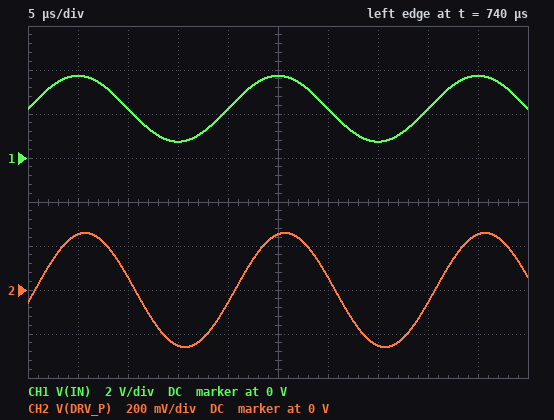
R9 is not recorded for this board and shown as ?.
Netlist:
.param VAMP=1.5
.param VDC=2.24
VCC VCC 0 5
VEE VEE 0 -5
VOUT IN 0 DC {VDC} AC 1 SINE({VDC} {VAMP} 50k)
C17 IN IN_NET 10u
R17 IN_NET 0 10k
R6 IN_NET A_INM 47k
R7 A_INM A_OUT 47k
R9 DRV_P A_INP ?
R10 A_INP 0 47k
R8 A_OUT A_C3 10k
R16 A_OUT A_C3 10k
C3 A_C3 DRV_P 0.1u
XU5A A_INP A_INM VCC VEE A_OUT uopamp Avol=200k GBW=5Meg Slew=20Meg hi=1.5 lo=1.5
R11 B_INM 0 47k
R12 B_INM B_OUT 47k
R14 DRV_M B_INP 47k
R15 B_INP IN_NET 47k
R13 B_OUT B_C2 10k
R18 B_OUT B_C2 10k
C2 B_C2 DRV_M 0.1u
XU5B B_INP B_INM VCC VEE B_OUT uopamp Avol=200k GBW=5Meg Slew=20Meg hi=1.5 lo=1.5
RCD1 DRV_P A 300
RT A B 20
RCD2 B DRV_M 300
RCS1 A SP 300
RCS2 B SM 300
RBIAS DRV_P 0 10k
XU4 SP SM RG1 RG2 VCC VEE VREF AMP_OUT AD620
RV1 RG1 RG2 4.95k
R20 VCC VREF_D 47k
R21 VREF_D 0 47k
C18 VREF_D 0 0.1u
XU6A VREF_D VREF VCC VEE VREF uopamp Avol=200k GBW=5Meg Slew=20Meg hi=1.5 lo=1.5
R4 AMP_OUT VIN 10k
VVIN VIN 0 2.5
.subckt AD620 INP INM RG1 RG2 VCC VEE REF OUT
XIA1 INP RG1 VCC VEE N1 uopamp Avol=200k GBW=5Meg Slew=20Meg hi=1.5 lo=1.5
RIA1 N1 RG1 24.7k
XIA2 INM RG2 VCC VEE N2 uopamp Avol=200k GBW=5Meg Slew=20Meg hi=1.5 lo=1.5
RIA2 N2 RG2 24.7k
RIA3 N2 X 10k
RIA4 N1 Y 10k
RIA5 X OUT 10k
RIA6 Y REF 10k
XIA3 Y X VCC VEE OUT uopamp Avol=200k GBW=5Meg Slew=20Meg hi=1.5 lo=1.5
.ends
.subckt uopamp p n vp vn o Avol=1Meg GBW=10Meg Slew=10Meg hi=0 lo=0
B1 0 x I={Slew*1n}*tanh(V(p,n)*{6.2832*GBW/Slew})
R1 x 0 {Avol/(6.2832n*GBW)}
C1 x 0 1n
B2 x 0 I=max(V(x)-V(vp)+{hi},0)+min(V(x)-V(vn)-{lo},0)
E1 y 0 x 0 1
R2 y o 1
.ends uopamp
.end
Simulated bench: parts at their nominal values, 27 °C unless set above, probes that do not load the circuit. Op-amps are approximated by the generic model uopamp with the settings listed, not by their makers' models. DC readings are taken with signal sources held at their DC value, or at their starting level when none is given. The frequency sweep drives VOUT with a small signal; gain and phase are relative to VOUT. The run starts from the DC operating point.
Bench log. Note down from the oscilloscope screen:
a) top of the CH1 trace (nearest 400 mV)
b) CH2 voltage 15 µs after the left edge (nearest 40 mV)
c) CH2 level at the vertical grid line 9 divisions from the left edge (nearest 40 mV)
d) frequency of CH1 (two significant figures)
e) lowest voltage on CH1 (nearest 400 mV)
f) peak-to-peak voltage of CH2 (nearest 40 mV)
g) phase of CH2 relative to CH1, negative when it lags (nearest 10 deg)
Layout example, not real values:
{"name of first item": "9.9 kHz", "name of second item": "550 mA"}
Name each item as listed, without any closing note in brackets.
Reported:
{"top of the CH1 trace": "3.6 V", "CH2 voltage 15 µs after the left edge": "-240 mV", "CH2 level at the vertical grid line 9 divisions from the left edge": "240 mV", "frequency of CH1": "50 kHz", "lowest voltage on CH1": "800 mV", "peak-to-peak voltage of CH2": "520 mV", "phase of CH2 relative to CH1, negative when it lags": "-10 deg"}
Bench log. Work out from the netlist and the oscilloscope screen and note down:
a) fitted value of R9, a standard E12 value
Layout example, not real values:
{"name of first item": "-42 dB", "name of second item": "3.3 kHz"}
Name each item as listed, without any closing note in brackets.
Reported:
{"fitted value of R9, a standard E12 value": "22 kΩ"}
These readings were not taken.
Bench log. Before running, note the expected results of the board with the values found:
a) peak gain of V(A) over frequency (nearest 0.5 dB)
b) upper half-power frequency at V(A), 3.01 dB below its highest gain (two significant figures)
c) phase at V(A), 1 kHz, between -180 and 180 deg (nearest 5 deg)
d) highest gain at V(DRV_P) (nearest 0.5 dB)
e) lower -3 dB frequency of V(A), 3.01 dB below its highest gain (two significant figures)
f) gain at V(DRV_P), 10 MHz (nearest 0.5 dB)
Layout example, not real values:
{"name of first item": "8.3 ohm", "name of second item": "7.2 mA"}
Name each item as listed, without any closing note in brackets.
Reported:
{"peak gain of V(A) over frequency": "-12.5 dB", "upper half-power frequency at V(A), 3.01 dB below its highest gain": "260 kHz", "phase at V(A), 1 kHz, between -180 and 180 deg": "15 deg", "highest gain at V(DRV_P)": "-15.0 dB", "lower -3 dB frequency of V(A), 3.01 dB below its highest gain": "470 Hz", "gain at V(DRV_P), 10 MHz": "-35.0 dB"}
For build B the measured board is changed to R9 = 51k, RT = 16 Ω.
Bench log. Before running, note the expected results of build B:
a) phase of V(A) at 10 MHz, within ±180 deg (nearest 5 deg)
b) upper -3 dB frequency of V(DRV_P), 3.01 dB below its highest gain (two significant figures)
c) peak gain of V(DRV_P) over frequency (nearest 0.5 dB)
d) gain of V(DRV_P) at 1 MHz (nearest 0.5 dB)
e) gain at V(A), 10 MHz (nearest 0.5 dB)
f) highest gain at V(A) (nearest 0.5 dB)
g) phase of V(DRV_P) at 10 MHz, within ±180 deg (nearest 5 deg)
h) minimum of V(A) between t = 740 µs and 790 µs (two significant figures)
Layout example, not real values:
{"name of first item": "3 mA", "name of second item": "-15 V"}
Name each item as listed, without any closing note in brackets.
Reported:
{"phase of V(A) at 10 MHz, within ±180 deg": "-15 deg", "upper -3 dB frequency of V(DRV_P), 3.01 dB below its highest gain": "330 kHz", "peak gain of V(DRV_P) over frequency": "-21.0 dB", "gain of V(DRV_P) at 1 MHz": "-30.5 dB", "gain at V(A), 10 MHz": "-33.0 dB", "highest gain at V(A)": "-17.5 dB", "phase of V(DRV_P) at 10 MHz, within ±180 deg": "25 deg", "minimum of V(A) between t = 740 µs and 790 µs": "-200 mV"}
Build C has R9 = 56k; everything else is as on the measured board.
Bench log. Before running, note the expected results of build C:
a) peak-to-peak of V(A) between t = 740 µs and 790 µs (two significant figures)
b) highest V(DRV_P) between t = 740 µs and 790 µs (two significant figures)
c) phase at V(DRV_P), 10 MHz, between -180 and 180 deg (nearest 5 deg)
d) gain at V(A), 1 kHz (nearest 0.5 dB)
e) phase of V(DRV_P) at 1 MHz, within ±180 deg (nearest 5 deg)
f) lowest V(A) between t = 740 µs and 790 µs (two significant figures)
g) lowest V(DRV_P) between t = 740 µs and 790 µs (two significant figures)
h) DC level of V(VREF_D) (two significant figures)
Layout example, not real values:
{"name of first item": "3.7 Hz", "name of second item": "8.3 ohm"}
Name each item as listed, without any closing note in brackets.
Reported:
{"peak-to-peak of V(A) between t = 740 µs and 790 µs": "390 mV", "highest V(DRV_P) between t = 740 µs and 790 µs": "100 mV", "phase at V(DRV_P), 10 MHz, between -180 and 180 deg": "25 deg", "gain at V(A), 1 kHz": "-18.0 dB", "phase of V(DRV_P) at 1 MHz, within ±180 deg": "-95 deg", "lowest V(A) between t = 740 µs and 790 µs": "-190 mV", "lowest V(DRV_P) between t = 740 µs and 790 µs": "-100 mV", "DC level of V(VREF_D)": "2.5 V"}
